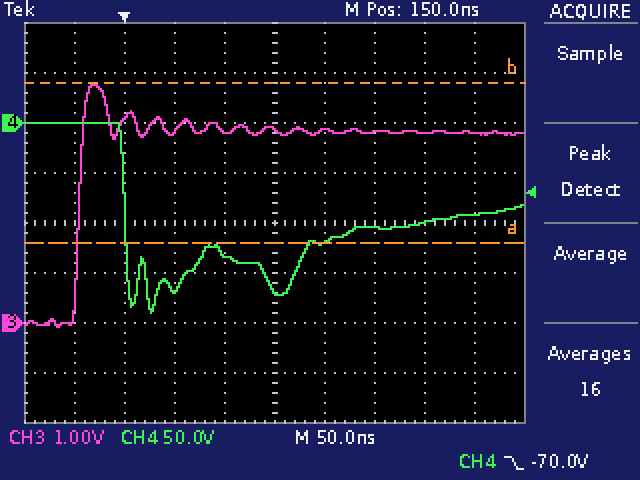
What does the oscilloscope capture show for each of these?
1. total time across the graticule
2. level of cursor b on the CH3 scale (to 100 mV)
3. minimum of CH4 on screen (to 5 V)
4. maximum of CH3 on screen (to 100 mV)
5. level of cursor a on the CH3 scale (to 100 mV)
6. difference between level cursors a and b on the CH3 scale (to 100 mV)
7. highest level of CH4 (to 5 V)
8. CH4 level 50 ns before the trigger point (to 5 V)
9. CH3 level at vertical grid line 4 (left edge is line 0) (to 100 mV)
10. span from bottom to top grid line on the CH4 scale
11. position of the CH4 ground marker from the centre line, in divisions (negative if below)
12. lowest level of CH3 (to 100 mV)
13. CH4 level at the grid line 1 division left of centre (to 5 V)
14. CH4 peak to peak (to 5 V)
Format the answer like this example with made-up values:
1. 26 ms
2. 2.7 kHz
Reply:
1. 500 ns
2. 4.8 V
3. -190 V
4. 4.8 V
5. 1.6 V
6. 3.2 V
7. 0 V
8. 0 V
9. 3.8 V
10. 400 V
11. +2.0 div
12. -100 mV
13. -130 V
14. 190 V
